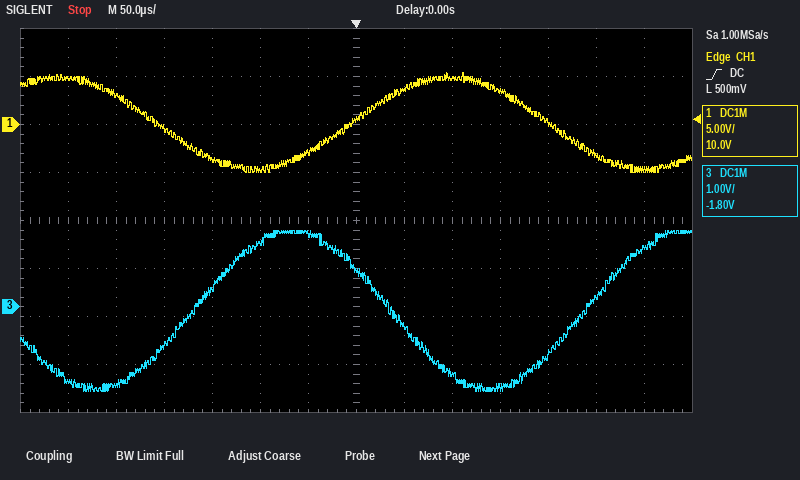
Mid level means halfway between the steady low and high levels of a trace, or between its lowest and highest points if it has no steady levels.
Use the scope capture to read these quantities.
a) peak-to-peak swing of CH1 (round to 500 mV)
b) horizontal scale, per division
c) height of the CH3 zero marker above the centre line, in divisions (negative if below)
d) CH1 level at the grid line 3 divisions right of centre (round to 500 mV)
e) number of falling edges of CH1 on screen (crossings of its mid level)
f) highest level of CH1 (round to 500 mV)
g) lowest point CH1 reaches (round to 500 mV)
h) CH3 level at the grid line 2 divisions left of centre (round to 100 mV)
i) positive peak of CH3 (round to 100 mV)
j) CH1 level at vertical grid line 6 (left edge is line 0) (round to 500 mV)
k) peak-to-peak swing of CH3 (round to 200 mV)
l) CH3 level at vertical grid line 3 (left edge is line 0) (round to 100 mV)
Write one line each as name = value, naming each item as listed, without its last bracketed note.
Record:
peak-to-peak swing of CH1 = 10.5 V
horizontal scale, per division = 50 µs
height of the CH3 zero marker above the centre line, in divisions = -1.8 div
CH1 level at the grid line 3 divisions right of centre = 3.5 V
number of falling edges of CH1 on screen = 2
highest level of CH1 = 5.5 V
lowest point CH1 reaches = -5.0 V
CH3 level at the grid line 2 divisions left of centre = 1.3 V
positive peak of CH3 = 1.6 V
CH1 level at vertical grid line 6 (left edge is line 0) = -3.0 V
peak-to-peak swing of CH3 = 3.4 V
CH3 level at vertical grid line 3 (left edge is line 0) = -800 mV
